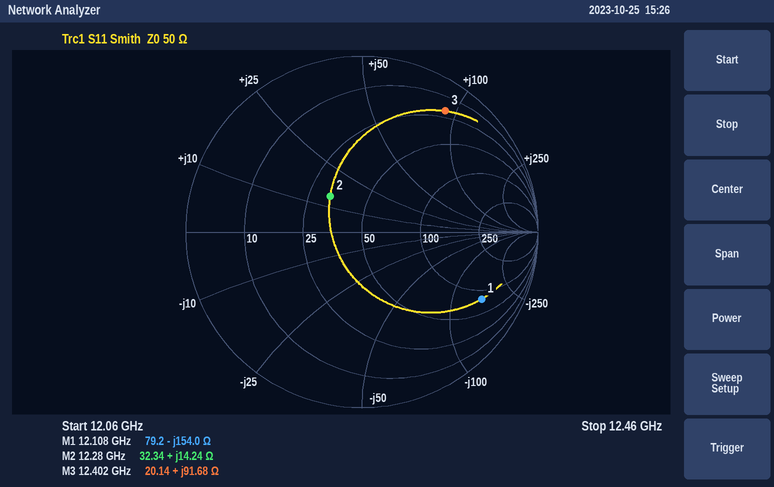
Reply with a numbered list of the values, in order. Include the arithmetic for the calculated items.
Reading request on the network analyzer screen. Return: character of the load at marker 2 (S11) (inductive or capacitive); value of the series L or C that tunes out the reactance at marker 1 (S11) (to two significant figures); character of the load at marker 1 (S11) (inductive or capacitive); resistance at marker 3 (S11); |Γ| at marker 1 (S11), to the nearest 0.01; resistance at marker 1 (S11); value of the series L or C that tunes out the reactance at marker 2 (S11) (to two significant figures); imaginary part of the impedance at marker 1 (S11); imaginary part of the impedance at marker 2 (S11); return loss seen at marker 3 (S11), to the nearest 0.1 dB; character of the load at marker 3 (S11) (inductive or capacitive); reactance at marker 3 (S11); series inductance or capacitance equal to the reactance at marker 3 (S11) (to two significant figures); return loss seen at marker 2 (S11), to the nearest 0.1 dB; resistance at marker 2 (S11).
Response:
1. inductive
2. L = 154 Ω/(2π × 12.108 GHz) ≈ 2.0 nH
3. capacitive
4. 20.14 Ω
5. 0.78
6. 79.2 Ω
7. C = 1/(2π × 12.28 GHz × 14.24 Ω) ≈ 910 fF
8. -154.0 Ω
9. +14.24 Ω
10. 1.6 dB
11. inductive
12. +91.68 Ω
13. L = 91.68 Ω/(2π × 12.402 GHz) ≈ 1.2 nH
14. 11.3 dB
15. 32.34 Ω
